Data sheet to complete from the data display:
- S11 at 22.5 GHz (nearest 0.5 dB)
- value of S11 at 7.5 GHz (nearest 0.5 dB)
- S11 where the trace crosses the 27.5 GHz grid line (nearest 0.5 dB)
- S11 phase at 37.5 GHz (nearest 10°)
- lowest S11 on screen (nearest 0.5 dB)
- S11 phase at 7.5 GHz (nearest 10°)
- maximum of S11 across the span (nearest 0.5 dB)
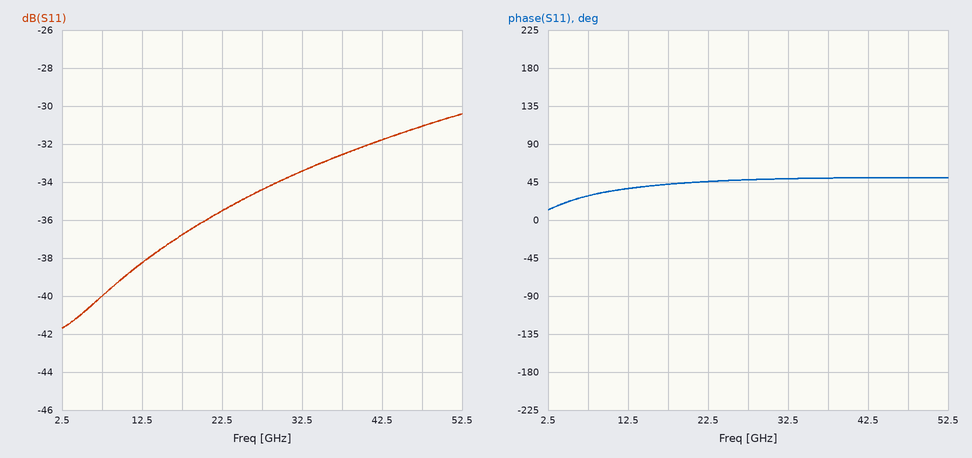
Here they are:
-35.5 dB
-40.0 dB
-34.5 dB
50°
-41.5 dB
30°
-30.5 dB
